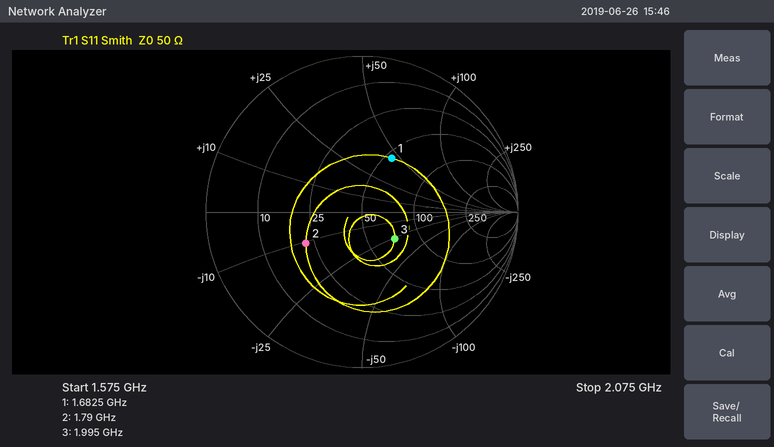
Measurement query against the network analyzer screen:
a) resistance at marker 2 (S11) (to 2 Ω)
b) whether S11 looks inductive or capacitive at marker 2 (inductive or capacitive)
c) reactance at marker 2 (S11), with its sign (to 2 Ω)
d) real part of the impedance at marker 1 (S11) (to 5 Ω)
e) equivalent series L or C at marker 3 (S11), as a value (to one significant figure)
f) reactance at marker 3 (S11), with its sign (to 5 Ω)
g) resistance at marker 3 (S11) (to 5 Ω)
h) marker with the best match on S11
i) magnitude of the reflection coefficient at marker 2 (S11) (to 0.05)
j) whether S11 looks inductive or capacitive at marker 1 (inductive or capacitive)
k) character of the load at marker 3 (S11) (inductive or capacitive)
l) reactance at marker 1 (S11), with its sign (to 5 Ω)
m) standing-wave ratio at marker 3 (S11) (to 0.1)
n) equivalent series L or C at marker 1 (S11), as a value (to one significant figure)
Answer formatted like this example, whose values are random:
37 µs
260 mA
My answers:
22 Ω
capacitive
-10 Ω
55 Ω
3 pF
-25 Ω
70 Ω
marker 3
0.40
inductive
capacitive
+45 Ω
1.7
4 nH
